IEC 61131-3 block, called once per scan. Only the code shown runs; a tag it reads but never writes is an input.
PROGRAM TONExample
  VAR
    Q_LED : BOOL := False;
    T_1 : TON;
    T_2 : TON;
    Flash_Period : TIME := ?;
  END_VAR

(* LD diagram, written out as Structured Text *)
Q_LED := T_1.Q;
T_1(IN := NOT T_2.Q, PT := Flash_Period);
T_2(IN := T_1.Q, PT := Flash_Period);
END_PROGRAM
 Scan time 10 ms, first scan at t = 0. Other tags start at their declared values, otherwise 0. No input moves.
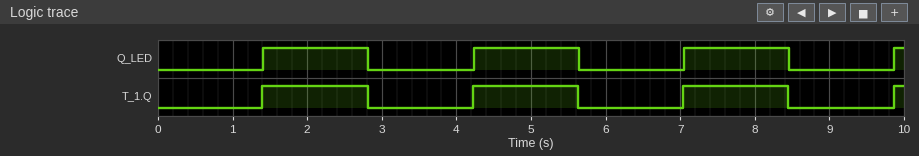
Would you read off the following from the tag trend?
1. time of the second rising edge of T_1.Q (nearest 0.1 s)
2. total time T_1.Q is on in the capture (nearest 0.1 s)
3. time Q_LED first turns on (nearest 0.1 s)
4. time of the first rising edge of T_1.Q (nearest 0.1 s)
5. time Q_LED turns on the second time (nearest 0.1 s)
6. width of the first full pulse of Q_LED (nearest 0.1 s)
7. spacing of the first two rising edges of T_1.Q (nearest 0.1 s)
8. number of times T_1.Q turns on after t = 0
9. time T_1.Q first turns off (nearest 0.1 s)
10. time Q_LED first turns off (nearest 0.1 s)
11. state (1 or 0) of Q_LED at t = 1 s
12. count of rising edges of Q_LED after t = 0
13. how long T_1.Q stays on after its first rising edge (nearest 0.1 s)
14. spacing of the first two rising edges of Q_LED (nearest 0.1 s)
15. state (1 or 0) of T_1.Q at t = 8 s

4.2 s
4.4 s
1.4 s
1.4 s
4.2 s
1.4 s
2.8 s
4
2.8 s
2.8 s
0
4
1.4 s
2.8 s
1
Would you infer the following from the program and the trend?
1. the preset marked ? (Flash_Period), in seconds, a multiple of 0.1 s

1.4 s
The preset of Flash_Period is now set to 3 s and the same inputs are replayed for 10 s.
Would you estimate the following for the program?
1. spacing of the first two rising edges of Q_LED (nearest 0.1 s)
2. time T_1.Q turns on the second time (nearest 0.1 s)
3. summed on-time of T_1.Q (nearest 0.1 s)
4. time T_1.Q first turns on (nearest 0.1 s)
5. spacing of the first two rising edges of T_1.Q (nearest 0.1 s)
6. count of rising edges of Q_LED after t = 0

6.0 s
9.0 s
4.0 s
3.0 s
6.0 s
2
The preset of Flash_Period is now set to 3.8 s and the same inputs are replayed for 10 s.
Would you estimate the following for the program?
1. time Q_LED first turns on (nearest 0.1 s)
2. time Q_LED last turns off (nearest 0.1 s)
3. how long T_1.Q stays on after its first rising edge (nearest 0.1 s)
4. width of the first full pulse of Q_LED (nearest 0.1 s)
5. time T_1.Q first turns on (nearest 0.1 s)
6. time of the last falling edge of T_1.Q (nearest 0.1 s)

3.8 s
7.6 s
3.8 s
3.8 s
3.8 s
7.6 s
